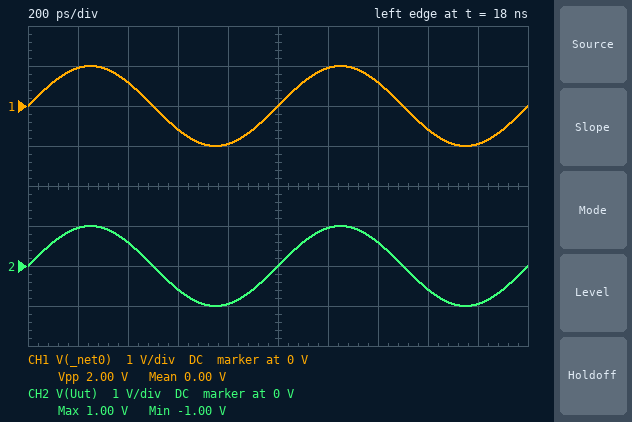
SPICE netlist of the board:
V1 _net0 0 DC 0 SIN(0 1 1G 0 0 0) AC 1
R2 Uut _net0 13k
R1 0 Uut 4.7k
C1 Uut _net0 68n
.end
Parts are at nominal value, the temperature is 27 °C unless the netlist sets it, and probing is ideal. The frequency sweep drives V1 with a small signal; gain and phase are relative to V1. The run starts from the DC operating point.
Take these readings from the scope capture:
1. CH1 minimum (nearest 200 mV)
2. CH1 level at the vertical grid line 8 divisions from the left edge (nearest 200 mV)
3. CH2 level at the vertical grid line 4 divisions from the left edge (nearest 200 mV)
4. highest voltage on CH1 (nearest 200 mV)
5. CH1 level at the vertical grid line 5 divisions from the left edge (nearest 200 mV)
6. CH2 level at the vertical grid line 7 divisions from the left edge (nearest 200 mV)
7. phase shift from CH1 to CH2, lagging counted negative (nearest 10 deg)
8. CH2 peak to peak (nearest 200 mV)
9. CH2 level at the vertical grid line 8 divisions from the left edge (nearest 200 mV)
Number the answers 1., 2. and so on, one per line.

1. -1.0 V
2. -600 mV
3. -1.0 V
4. 1.0 V
5. 0 V
6. 600 mV
7. 0 deg
8. 2.0 V
9. -600 mV
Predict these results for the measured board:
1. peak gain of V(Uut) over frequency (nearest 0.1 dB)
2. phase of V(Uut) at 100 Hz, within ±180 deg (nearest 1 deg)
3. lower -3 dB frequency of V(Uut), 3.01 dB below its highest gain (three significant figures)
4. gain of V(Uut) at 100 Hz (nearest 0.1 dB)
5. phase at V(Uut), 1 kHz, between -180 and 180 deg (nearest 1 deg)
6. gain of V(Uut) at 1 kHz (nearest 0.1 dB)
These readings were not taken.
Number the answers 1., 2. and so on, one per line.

1. 0 dB
2. 21 deg
3. 628 Hz
4. -10.4 dB
5. 24 deg
6. -1.5 dB
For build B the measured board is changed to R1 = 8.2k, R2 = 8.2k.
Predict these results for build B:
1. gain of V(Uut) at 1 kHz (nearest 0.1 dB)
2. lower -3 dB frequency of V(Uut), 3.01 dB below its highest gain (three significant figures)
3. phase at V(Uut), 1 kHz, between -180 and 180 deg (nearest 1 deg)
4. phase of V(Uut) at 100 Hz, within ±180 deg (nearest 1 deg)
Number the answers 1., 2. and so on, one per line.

1. -0.9 dB
2. 404 Hz
3. 14 deg
4. 9 deg
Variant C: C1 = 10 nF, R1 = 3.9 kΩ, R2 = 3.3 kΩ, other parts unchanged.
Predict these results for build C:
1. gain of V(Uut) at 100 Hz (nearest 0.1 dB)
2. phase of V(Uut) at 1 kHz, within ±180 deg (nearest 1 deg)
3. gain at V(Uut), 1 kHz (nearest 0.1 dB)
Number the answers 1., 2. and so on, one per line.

1. -5.3 dB
2. 5 deg
3. -5.2 dB
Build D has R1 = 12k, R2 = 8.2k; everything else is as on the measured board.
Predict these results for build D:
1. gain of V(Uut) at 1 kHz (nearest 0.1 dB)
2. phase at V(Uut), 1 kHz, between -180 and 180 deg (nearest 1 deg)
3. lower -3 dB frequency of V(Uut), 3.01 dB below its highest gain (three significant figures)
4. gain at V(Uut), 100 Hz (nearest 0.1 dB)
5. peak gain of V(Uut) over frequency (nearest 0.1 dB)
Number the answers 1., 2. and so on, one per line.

1. -0.6 dB
2. 10 deg
3. 261 Hz
4. -4.2 dB
5. 0 dB
